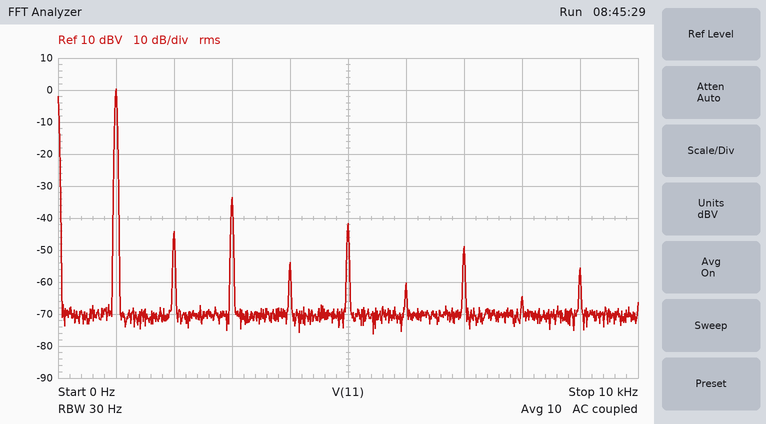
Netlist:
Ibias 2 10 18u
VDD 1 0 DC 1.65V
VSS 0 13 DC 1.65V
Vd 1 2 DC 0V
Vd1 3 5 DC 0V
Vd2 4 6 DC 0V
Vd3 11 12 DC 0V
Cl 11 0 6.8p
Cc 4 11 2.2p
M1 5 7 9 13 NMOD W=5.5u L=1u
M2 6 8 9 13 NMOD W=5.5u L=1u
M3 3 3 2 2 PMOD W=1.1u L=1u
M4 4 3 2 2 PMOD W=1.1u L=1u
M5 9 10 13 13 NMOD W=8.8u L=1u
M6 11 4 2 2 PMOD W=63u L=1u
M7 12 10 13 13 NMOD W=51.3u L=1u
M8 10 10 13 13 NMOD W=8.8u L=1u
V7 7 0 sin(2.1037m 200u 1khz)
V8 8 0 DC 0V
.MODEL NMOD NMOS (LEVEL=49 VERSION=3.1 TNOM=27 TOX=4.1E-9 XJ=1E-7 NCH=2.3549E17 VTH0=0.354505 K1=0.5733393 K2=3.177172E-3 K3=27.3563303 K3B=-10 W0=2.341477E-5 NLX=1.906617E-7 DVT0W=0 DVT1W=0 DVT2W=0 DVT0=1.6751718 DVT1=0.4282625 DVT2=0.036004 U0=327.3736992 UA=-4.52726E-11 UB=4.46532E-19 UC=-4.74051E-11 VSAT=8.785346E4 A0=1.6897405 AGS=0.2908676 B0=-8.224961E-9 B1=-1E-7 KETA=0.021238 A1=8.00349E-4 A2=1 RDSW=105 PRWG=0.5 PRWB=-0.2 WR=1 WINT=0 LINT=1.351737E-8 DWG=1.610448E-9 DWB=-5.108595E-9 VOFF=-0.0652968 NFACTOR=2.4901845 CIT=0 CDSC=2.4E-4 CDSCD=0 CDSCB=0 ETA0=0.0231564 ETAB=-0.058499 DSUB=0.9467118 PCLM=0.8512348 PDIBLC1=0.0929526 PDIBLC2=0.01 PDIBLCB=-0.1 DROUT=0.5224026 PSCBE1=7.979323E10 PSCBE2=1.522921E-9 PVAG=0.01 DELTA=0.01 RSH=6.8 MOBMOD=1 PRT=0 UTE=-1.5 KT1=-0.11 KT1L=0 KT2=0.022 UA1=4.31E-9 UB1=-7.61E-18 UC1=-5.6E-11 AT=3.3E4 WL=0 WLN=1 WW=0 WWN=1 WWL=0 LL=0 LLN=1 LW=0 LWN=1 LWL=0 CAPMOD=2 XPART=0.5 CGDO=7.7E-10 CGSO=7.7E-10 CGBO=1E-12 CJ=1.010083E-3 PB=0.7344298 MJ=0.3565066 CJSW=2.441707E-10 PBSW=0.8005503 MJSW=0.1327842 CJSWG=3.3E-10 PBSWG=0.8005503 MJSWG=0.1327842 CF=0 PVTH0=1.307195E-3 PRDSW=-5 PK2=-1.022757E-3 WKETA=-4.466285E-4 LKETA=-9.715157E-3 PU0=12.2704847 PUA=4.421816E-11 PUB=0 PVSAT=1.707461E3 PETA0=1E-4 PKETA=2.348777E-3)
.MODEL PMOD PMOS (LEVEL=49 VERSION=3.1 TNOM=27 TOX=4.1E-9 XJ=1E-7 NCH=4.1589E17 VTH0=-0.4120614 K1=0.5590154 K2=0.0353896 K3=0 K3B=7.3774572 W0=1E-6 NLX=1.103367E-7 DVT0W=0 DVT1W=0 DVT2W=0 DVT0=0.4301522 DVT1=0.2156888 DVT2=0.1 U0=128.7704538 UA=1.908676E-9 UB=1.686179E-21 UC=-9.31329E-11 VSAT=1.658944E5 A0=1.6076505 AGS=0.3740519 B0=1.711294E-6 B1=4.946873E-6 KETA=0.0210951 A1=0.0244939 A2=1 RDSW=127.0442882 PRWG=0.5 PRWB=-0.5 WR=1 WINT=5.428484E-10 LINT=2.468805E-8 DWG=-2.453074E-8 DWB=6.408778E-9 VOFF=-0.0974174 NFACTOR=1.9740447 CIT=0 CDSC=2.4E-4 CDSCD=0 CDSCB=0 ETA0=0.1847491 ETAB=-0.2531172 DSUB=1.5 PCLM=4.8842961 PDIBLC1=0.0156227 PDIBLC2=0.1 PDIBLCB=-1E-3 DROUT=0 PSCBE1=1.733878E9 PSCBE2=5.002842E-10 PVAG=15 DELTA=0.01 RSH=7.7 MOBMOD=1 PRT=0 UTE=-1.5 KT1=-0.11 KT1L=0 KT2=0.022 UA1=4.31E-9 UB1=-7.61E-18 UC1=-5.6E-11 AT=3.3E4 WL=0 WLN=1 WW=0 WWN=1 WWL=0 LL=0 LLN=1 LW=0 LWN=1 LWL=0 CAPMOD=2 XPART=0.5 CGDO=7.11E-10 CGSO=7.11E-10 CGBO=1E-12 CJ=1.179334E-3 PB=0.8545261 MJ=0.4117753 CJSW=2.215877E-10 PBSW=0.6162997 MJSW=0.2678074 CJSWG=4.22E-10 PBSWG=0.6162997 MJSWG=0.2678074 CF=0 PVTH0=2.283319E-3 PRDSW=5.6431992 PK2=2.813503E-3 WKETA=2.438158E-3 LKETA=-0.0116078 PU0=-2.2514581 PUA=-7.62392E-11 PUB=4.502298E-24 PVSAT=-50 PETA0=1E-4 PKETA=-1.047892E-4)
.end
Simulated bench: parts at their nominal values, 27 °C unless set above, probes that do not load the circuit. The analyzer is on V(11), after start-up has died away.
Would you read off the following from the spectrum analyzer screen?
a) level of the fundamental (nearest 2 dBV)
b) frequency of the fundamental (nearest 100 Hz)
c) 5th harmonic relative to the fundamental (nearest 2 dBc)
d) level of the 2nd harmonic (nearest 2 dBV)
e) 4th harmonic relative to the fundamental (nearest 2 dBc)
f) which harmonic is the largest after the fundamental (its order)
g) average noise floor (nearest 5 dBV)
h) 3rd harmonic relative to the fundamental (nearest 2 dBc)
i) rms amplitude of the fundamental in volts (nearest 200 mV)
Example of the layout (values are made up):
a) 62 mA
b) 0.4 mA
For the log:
a) 0 dBV
b) 1.0 kHz
c) -42 dBc
d) -44 dBV
e) -54 dBc
f) 3
g) -70 dBV
h) -34 dBc
i) 1.0 V
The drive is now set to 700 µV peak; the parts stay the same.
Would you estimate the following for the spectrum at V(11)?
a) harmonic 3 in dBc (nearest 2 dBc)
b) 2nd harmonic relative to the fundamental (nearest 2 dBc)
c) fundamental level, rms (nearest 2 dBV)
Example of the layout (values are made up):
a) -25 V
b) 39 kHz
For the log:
a) -12 dBc
b) -48 dBc
c) 2 dBV
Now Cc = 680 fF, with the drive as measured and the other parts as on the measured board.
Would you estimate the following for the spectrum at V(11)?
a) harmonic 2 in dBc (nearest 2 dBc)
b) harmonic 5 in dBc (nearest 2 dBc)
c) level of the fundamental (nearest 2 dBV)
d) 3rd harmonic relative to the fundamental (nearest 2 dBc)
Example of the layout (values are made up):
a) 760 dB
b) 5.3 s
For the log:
a) -42 dBc
b) -34 dBc
c) 2 dBV
d) -18 dBc
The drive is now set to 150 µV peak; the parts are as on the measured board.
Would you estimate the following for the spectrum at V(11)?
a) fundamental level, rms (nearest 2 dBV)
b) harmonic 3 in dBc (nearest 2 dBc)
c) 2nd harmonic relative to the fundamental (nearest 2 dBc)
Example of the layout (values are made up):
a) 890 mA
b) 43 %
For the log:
a) -2 dBV
b) -58 dBc
c) -60 dBc
